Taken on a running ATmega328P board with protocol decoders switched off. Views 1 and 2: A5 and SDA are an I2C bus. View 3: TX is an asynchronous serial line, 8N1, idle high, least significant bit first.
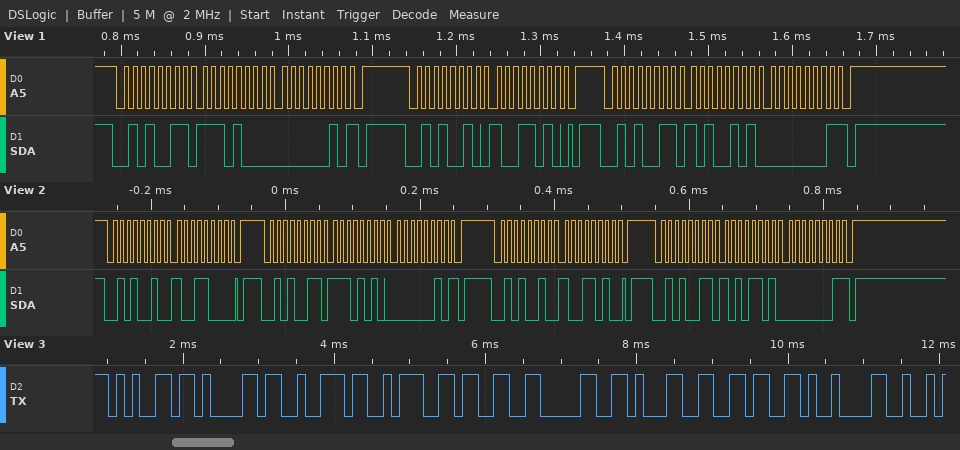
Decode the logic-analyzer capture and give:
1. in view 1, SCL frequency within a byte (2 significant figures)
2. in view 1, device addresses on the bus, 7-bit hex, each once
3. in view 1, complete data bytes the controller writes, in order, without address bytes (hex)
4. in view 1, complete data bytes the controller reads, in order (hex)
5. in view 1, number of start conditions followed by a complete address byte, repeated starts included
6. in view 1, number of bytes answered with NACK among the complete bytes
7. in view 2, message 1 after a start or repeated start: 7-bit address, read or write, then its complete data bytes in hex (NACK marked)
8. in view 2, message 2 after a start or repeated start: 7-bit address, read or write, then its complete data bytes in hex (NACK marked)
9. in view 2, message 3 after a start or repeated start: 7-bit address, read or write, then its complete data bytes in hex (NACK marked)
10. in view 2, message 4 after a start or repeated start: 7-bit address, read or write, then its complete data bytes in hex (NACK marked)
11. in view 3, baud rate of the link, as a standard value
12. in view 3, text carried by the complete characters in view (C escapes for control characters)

100 kHz
0x29
9A
E8 02 A5 01
3
2
0x29 write: 98
0x29 read: EA 02 NACK
0x29 write: 9A
0x29 read: AD 01 NACK
9600 baud
"ear:3016\t"
